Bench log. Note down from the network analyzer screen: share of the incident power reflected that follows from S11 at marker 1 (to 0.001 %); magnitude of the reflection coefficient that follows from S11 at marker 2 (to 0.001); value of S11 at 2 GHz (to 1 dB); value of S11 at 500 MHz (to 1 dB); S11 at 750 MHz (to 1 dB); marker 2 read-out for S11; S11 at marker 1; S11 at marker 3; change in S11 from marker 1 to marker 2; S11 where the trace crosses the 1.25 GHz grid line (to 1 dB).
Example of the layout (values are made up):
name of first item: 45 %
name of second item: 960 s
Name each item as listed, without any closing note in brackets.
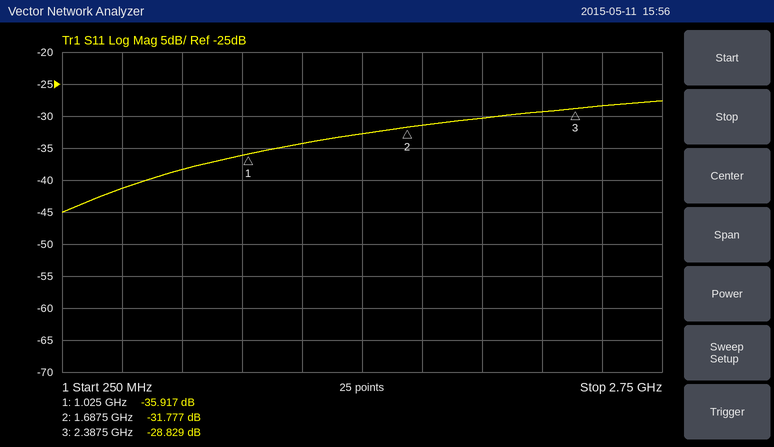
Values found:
share of the incident power reflected that follows from S11 at marker 1: 0.026 %
magnitude of the reflection coefficient that follows from S11 at marker 2: 0.026
value of S11 at 2 GHz: -30 dB
value of S11 at 500 MHz: -41 dB
S11 at 750 MHz: -38 dB
marker 2 read-out for S11: -31.777 dB
S11 at marker 1: -35.917 dB
S11 at marker 3: -28.829 dB
change in S11 from marker 1 to marker 2: 4.140 dB
S11 where the trace crosses the 1.25 GHz grid line: -34 dB
